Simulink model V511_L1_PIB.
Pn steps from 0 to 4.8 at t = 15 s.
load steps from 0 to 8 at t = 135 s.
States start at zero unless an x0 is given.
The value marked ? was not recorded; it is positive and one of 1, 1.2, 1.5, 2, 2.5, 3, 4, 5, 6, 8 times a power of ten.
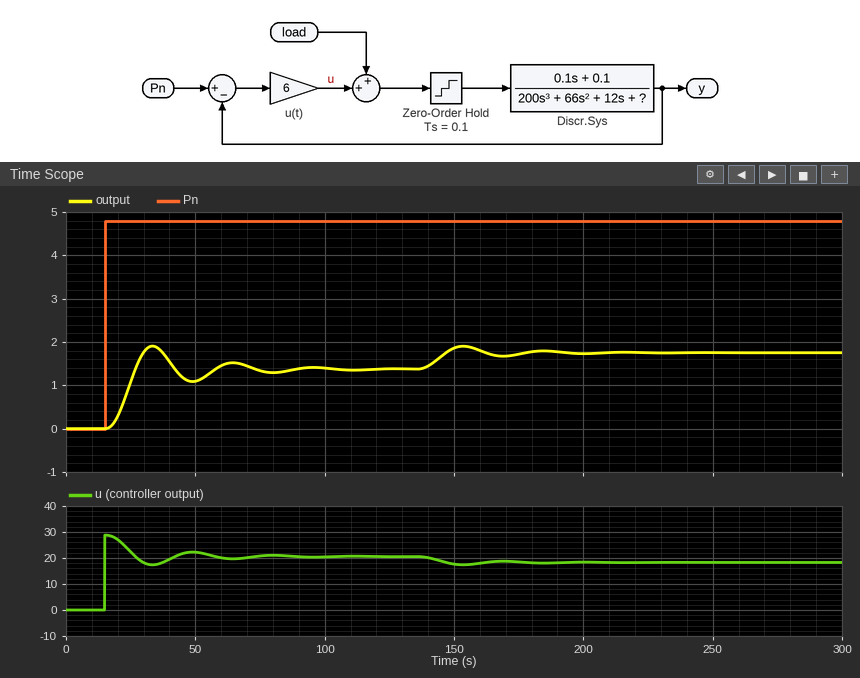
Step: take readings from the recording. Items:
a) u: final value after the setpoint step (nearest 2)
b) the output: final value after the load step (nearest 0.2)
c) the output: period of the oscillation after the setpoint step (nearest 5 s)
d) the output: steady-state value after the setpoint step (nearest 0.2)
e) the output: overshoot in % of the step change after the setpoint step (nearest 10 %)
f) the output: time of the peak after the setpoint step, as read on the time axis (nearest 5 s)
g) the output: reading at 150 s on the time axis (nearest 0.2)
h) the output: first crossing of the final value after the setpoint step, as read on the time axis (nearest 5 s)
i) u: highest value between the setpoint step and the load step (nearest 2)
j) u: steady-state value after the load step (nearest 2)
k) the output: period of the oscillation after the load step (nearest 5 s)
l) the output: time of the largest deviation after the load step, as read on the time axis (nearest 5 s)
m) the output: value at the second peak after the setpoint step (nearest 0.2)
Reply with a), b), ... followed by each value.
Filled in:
a) 20
b) 1.8
c) 30 s
d) 1.4
e) 40 %
f) 35 s
g) 1.8
h) 25 s
i) 28
j) 18
k) 30 s
l) 155 s
m) 1.6
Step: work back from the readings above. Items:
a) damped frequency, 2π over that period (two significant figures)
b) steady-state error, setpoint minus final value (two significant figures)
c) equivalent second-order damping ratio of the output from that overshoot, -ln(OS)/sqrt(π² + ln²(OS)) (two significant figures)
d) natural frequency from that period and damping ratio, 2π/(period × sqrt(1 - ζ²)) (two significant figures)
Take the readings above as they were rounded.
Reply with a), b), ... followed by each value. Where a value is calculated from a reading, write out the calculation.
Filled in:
a) 2π / 30 = 0.21 rad/s
b) 4.8 - 1.4 = 3.4
c) ln(0.4) = -0.916; 0.916 / sqrt(9.870 + 0.840) = 0.28
d) 2π / (30 × sqrt(1 - 0.28²)) = 0.22 rad/s
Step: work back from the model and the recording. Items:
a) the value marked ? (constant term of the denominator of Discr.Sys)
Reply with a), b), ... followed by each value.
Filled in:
a) 1.5
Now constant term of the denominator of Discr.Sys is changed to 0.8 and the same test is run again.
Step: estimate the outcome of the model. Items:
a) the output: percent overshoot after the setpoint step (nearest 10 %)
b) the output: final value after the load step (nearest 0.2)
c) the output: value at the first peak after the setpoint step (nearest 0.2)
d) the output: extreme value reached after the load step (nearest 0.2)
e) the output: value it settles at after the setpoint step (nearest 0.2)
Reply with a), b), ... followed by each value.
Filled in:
a) 20 %
b) 2.6
c) 2.4
d) 2.8
e) 2.0
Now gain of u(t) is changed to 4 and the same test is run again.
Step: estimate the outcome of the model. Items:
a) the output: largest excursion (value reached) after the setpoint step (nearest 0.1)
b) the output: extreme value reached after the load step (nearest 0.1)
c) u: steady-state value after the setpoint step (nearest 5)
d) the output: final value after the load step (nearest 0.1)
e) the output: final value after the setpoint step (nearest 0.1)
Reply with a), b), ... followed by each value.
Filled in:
a) 1.4
b) 1.6
c) 15
d) 1.4
e) 1.0
